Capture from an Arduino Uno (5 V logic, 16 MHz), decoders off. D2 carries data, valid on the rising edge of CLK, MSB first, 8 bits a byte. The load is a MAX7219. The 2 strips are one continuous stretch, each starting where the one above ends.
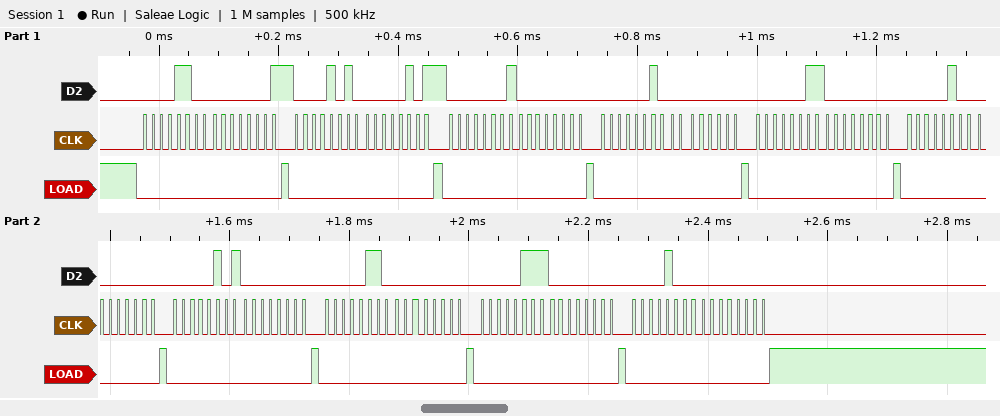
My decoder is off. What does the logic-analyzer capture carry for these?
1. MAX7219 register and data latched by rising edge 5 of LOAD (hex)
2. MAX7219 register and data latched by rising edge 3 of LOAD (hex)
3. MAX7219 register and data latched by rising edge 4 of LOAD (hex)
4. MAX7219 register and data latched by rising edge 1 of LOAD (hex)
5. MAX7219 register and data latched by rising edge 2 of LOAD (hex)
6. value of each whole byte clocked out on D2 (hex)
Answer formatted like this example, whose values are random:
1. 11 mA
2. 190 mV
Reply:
1. register 0x3, data 0x00
2. register 0x1, data 0x00
3. register 0x2, data 0x00
4. register 0xC, data 0x01
5. register 0xA, data 0x05
6. 0x0C 0x01 0x0A 0x05 0x01 0x00 0x02 0x00 0x03 0x00 0x04 0x00 0x05 0x00 0x06 0x00 0x07 0x00 0x08 0x00
